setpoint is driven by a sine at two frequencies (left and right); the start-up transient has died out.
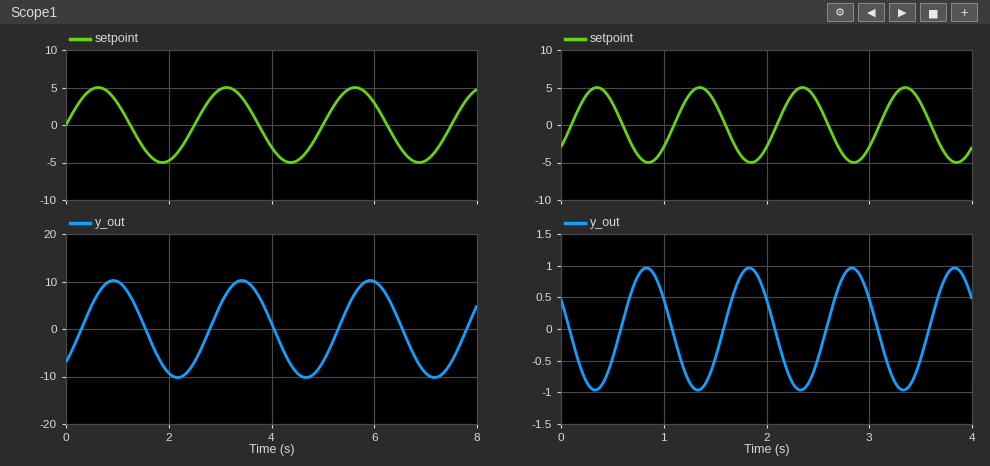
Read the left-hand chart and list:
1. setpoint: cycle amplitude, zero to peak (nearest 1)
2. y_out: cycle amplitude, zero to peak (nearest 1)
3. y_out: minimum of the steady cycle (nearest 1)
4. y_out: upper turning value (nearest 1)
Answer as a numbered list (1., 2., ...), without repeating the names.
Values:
1. 5
2. 10
3. -10
4. 10
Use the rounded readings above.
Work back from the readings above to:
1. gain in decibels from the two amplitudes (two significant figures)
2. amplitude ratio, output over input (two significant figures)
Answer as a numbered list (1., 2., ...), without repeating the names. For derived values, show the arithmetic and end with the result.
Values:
1. 20 log10(10 / 5) = 6.0 dB
2. 10 / 5 = 2.0
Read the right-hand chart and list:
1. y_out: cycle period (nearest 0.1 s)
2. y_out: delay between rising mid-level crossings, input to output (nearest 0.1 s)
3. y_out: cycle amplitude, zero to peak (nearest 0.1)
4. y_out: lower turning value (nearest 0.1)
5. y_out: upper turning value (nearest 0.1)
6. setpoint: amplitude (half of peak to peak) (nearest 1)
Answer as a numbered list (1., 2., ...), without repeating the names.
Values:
1. 1.0 s
2. 0.5 s
3. 1.0
4. -1.0
5. 1.0
6. 5
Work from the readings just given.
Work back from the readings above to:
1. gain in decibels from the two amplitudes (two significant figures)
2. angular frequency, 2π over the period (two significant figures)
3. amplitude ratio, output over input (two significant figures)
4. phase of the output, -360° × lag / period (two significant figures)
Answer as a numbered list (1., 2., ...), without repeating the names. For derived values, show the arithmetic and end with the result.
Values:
1. 20 log10(1 / 5) = -14 dB
2. 2π / 1 = 6.3 rad/s
3. 1 / 5 = 0.20
4. -360 × 0.5 / 1 = -180°
